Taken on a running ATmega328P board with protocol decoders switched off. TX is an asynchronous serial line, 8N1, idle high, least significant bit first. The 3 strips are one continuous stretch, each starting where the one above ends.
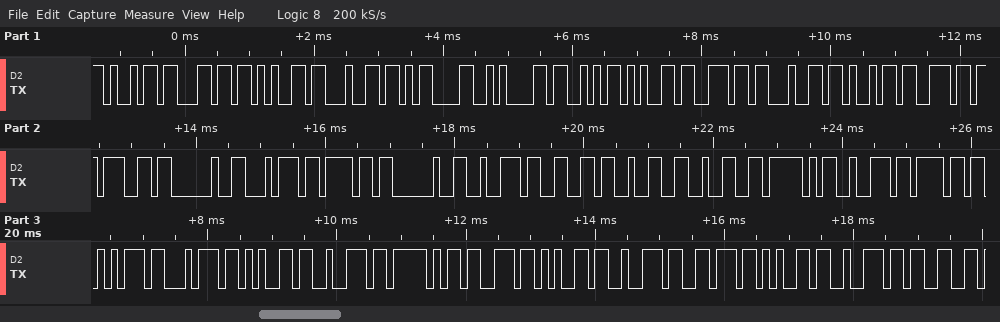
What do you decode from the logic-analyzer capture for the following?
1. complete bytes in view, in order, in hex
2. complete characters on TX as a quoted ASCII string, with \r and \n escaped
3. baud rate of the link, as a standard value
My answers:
0x69 0x6C 0x65 0x64 0x0D 0x0A 0x53 0x65 0x6E 0x64 0x69 0x6E 0x67 0x20 0x74 0x6F 0x20 0x72 0x66 0x32 0x32 0x5F 0x72 0x6F 0x75 0x74 0x65 0x72 0x5F 0x73 0x65 0x72 0x76 0x65 0x72 0x33
"iled\r\nSending to rf22_router_server3"
9600 baud
